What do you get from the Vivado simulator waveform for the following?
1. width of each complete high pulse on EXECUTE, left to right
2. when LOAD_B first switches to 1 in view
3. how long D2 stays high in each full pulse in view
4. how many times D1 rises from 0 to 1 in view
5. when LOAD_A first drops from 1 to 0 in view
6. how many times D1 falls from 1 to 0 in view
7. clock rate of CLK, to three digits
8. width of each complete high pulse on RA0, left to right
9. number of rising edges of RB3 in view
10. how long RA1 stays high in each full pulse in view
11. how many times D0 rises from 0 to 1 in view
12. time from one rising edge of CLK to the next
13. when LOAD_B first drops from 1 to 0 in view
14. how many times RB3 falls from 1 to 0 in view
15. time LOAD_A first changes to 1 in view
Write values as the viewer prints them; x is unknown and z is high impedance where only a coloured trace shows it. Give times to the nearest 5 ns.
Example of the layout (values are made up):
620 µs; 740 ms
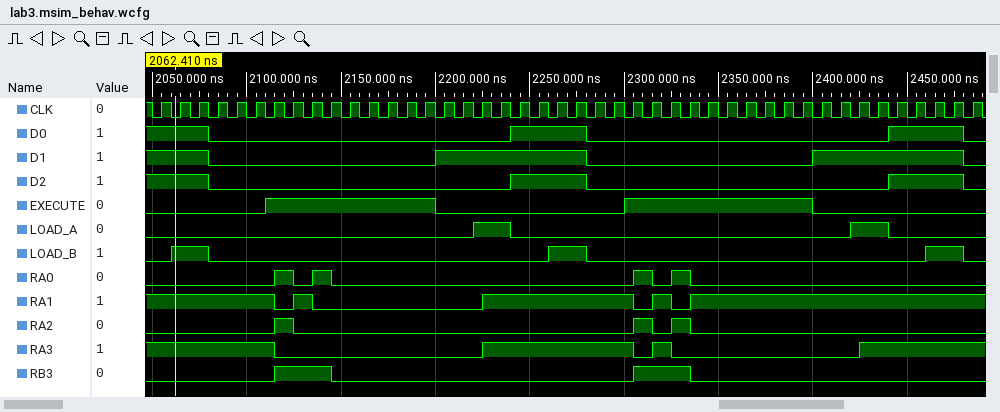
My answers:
90 ns, 100 ns; 2060 ns; 40 ns, 40 ns; 2; 2240 ns; 3; 100 MHz; 10 ns, 10 ns, 10 ns, 10 ns; 2; 10 ns, 80 ns, 10 ns; 2; 10 ns; 2080 ns; 2; 2220 ns
